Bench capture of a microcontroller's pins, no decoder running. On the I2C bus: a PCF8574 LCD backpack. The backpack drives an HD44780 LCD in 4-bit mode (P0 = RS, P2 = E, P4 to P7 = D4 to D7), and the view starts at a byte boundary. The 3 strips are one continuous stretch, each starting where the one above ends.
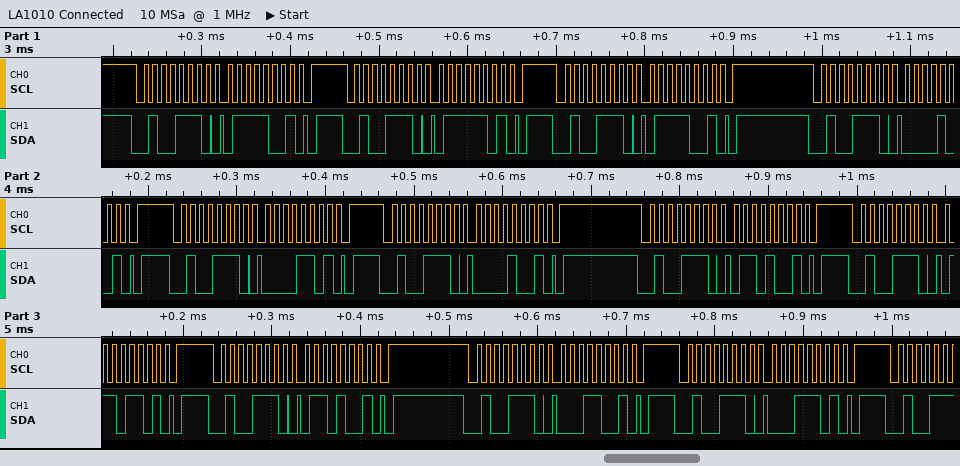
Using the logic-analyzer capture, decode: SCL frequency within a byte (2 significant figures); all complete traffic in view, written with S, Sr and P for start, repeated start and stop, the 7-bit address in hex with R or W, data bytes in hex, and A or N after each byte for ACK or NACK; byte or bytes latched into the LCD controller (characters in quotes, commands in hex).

100 kHz
S 27W A 79 A P S 27W A 7D A P S 27W A 79 A P S 27W A 09 A P S 27W A 0D A P S 27W A 09 A P S 27W A 69 A P S 27W A 6D A P S 27W A 69 A P S 27W A 19 A P S 27W A 1D A P
'p'
